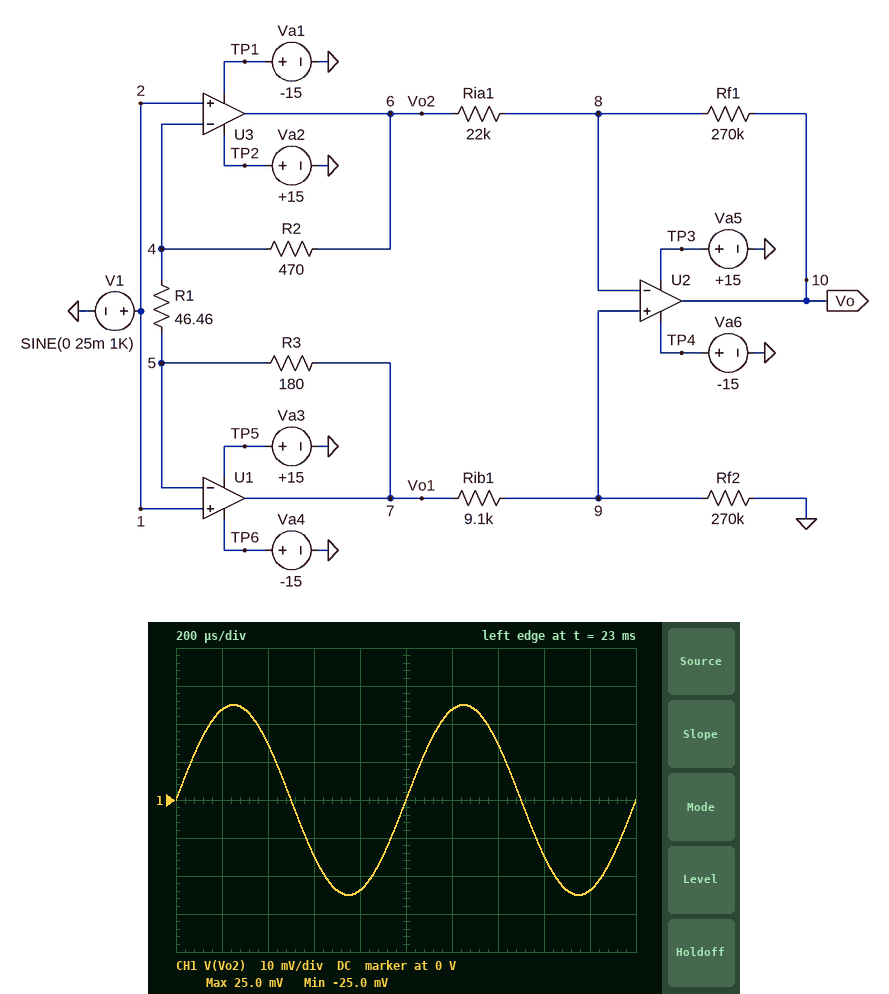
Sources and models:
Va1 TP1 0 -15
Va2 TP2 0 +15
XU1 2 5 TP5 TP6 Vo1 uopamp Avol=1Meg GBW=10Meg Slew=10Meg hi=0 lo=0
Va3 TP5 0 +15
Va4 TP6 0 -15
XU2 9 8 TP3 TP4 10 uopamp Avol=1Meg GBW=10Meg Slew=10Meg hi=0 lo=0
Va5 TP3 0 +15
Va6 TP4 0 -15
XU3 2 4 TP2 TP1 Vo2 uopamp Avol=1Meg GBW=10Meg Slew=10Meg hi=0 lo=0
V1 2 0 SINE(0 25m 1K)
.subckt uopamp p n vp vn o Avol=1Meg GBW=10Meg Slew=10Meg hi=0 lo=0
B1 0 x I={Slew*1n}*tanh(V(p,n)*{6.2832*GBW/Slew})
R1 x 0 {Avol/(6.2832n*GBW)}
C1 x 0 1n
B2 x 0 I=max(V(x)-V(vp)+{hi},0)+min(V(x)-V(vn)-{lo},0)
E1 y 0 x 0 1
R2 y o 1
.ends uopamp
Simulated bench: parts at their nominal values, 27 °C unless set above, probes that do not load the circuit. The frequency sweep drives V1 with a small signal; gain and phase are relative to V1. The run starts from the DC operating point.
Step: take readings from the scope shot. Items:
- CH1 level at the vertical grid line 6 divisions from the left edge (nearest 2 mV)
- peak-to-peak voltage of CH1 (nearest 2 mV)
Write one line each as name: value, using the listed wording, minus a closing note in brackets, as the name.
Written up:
CH1 level at the vertical grid line 6 divisions from the left edge: 24 mV
peak-to-peak voltage of CH1: 50 mV
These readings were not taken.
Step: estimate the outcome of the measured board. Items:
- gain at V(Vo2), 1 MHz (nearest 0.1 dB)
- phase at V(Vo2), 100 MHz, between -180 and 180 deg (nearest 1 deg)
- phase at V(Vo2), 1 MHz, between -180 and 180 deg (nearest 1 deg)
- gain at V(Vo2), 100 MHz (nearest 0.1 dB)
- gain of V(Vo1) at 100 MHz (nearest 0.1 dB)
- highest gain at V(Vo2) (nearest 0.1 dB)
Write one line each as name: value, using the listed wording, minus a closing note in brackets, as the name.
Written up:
gain at V(Vo2), 1 MHz: 0 dB
phase at V(Vo2), 100 MHz, between -180 and 180 deg: -84 deg
phase at V(Vo2), 1 MHz, between -180 and 180 deg: -6 deg
gain at V(Vo2), 100 MHz: -20.0 dB
gain of V(Vo1) at 100 MHz: -20.0 dB
highest gain at V(Vo2): 0 dB
